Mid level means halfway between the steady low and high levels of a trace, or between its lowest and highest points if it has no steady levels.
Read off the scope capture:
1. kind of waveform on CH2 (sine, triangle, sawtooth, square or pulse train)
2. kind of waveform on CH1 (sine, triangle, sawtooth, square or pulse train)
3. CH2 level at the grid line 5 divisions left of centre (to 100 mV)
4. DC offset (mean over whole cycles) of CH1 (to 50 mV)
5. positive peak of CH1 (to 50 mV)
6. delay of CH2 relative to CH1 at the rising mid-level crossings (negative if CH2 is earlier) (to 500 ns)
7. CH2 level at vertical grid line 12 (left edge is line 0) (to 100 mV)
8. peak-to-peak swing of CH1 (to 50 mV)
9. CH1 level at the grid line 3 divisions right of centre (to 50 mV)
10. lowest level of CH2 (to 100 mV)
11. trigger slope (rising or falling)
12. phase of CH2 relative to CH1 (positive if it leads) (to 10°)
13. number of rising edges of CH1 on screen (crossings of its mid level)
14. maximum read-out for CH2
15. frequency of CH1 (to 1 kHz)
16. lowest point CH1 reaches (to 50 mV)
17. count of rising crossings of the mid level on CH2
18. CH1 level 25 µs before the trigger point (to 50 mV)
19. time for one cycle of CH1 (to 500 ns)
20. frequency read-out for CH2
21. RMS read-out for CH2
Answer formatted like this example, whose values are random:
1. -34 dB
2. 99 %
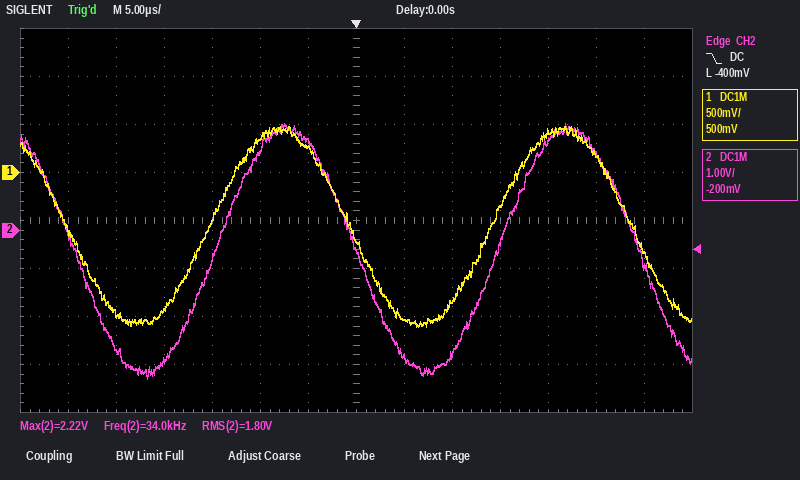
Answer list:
1. sine
2. sine
3. -2.5 V
4. -550 mV
5. 500 mV
6. +500 ns
7. 1.6 V
8. 2.10 V
9. -350 mV
10. -3.1 V
11. falling
12. -10°
13. 2
14. 2.22 V
15. 34 kHz
16. -1.60 V
17. 2
18. -1.45 V
19. 29.5 µs
20. 34.0 kHz
21. 1.80 V
